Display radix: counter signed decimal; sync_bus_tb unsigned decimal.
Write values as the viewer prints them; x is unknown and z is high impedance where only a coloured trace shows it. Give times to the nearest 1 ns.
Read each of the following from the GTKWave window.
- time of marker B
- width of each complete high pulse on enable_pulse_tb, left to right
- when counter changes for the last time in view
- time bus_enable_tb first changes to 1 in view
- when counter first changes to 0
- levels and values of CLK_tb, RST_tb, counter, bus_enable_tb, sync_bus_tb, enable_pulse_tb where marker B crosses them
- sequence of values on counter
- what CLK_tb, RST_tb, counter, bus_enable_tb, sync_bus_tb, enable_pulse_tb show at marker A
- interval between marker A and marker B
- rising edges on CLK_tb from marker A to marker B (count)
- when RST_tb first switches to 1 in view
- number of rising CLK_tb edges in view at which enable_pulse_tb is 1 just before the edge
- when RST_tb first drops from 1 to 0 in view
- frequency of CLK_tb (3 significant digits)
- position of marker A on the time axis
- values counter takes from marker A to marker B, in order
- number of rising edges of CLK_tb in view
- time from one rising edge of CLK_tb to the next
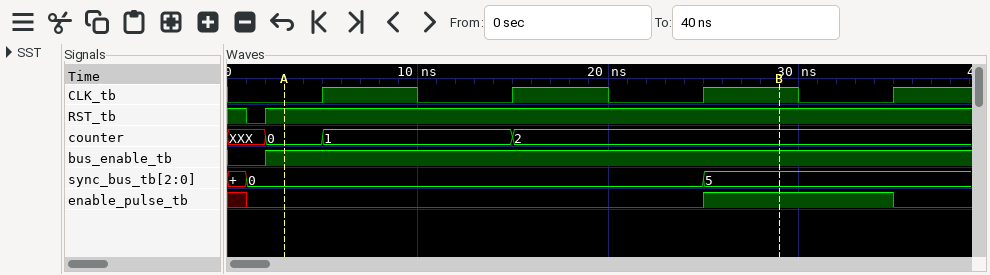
29 ns
10 ns
15 ns
2 ns
2 ns
CLK_tb=1, RST_tb=1, counter=2, bus_enable_tb=1, sync_bus_tb=5, enable_pulse_tb=1
XXX, 0, 1, 2
CLK_tb=0, RST_tb=1, counter=0, bus_enable_tb=1, sync_bus_tb=0, enable_pulse_tb=0
26 ns
3
2 ns
1
1 ns
100 MHz
3 ns
0, 1, 2
4
10 ns
